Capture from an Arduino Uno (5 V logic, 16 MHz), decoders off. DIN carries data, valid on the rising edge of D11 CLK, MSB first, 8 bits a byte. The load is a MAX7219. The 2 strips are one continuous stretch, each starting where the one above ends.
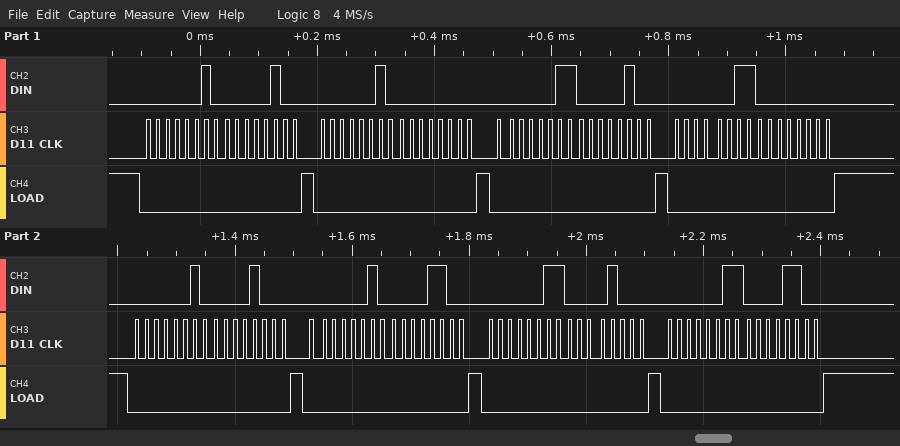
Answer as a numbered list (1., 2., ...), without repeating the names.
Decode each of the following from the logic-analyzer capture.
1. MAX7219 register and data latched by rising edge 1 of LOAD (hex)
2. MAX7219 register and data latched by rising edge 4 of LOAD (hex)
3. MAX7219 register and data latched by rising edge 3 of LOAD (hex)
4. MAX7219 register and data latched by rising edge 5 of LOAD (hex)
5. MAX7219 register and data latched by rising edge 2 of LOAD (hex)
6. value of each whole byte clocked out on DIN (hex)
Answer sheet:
1. register 0x2, data 0x04
2. register 0x3, data 0x00
3. register 0x3, data 0x04
4. register 0x2, data 0x08
5. register 0x2, data 0x00
6. 0x02 0x04 0x02 0x00 0x03 0x04 0x03 0x00 0x02 0x08 0x02 0x0C 0x03 0x08 0x03 0x0C
